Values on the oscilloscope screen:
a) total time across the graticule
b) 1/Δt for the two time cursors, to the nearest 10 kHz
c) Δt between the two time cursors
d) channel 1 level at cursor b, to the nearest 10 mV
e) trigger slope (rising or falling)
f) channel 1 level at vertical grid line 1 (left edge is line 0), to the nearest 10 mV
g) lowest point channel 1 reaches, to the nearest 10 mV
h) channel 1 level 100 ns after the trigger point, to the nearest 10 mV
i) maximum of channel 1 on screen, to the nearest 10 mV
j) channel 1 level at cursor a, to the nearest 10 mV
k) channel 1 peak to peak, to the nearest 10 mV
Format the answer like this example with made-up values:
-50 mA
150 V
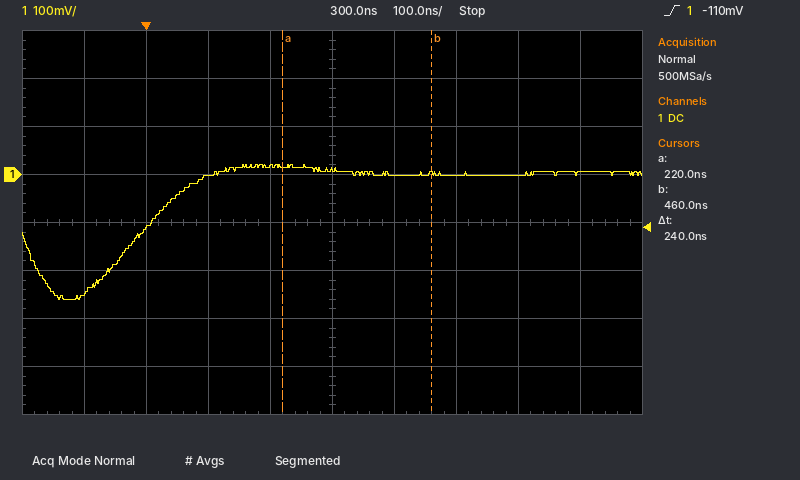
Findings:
1 µs
4.17 MHz
240 ns
0 mV
rising
-250 mV
-260 mV
0 mV
20 mV
20 mV
280 mV
